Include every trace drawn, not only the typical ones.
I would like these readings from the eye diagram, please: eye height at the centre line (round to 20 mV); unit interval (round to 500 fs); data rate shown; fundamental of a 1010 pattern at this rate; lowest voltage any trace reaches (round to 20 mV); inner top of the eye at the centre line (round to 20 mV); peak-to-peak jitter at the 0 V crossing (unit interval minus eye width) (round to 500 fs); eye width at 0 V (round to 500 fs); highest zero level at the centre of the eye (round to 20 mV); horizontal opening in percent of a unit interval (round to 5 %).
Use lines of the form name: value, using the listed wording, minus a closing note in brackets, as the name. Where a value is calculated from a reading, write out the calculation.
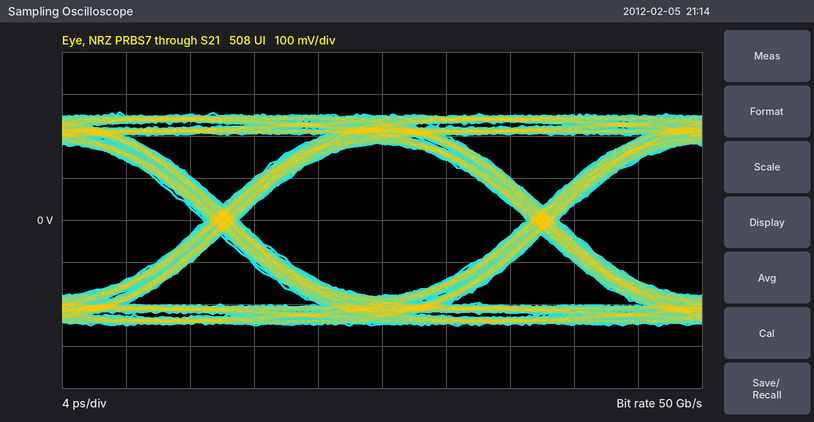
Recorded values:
eye height at the centre line: 360 mV
unit interval: 20.0 ps
data rate shown: 50 Gb/s
fundamental of a 1010 pattern at this rate: 25 GHz
lowest voltage any trace reaches: -260 mV
inner top of the eye at the centre line: 180 mV
peak-to-peak jitter at the 0 V crossing (unit interval minus eye width): 2.0 ps
eye width at 0 V: 18.0 ps
highest zero level at the centre of the eye: -180 mV
horizontal opening in percent of a unit interval: 18.0 ps / 20.0 ps ≈ 90 %
